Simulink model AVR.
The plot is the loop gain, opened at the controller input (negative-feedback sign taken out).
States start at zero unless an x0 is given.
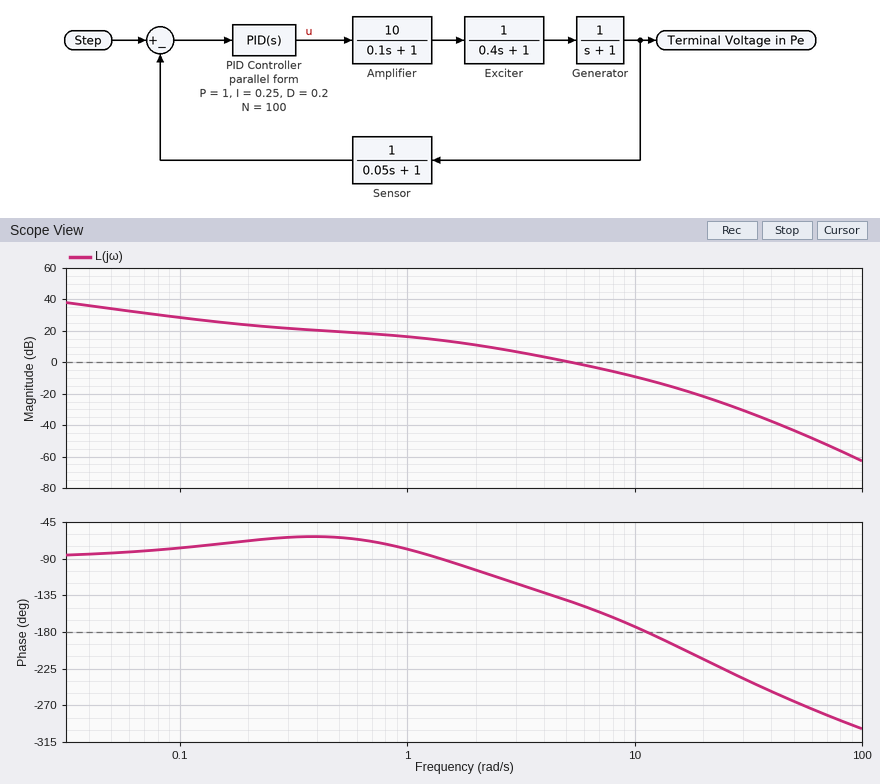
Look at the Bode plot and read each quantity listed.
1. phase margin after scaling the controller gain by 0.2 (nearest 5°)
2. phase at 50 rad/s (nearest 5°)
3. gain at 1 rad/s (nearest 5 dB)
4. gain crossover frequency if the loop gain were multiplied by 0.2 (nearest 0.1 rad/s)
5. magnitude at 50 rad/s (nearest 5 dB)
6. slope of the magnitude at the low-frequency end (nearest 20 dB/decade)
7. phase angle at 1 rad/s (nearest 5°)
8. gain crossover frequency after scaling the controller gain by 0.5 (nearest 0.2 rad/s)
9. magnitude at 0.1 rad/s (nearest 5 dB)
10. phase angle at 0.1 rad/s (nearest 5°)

90°
-265°
15 dB
1.4 rad/s
-45 dB
-20 dB/decade
-80°
3.2 rad/s
30 dB
-75°
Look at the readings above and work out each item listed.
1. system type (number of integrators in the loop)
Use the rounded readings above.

1
